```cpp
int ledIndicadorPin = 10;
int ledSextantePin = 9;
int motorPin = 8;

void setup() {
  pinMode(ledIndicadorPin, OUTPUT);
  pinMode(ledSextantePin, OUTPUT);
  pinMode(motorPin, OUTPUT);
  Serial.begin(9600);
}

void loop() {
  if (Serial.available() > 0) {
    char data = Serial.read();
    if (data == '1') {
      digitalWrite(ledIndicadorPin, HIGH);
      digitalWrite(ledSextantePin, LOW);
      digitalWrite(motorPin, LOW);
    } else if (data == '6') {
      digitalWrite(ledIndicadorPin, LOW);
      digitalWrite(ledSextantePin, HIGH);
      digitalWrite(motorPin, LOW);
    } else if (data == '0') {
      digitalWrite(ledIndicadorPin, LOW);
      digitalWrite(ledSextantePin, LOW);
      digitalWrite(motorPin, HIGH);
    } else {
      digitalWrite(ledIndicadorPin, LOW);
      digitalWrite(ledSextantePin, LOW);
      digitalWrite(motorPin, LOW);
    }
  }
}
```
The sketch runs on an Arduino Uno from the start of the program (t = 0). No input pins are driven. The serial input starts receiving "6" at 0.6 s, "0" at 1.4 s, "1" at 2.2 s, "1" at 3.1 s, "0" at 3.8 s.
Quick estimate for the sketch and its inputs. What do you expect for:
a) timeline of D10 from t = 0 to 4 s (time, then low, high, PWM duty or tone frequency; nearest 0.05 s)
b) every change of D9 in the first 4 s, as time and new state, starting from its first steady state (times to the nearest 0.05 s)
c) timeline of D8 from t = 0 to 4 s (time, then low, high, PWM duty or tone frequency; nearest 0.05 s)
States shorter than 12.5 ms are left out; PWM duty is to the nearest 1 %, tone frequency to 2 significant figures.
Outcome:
0 s low; 2.2 s high; 3.8 s low
0 s low; 0.6 s high; 1.4 s low
0 s low; 1.4 s high; 2.2 s low; 3.8 s high
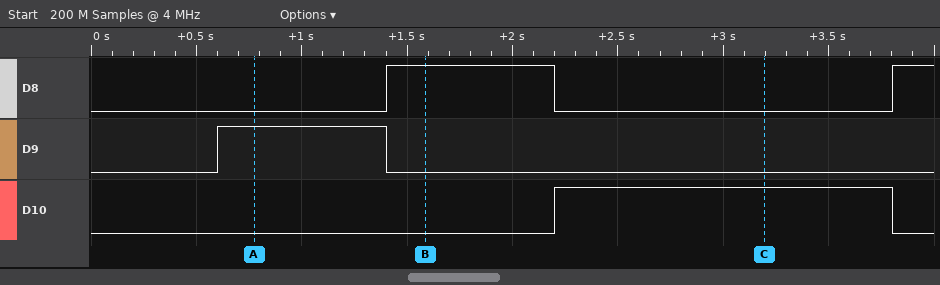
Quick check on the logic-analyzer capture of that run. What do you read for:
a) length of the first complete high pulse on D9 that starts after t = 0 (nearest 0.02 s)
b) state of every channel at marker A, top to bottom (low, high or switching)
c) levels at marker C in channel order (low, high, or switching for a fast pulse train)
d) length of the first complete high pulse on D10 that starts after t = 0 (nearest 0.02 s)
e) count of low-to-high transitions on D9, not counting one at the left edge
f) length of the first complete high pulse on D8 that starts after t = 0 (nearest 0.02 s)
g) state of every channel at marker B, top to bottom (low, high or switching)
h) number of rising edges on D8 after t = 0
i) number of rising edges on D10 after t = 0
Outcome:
0.80 s
D8 low, D9 high, D10 low
D8 low, D9 low, D10 high
1.60 s
1
0.80 s
D8 high, D9 low, D10 low
2
1
